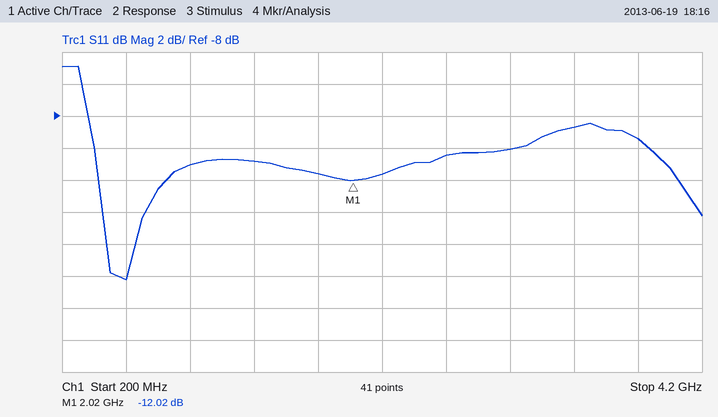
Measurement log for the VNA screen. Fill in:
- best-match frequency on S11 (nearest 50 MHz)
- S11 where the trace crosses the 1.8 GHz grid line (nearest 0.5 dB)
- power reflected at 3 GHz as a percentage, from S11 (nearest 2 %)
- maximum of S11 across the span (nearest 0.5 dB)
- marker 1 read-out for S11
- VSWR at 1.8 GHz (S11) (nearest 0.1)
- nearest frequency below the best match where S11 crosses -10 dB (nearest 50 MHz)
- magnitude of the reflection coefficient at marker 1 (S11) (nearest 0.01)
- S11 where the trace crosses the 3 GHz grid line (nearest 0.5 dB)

600 MHz
-11.5 dB
10 %
-5.0 dB
-12.02 dB
1.7
400 MHz
0.25
-10.0 dB
